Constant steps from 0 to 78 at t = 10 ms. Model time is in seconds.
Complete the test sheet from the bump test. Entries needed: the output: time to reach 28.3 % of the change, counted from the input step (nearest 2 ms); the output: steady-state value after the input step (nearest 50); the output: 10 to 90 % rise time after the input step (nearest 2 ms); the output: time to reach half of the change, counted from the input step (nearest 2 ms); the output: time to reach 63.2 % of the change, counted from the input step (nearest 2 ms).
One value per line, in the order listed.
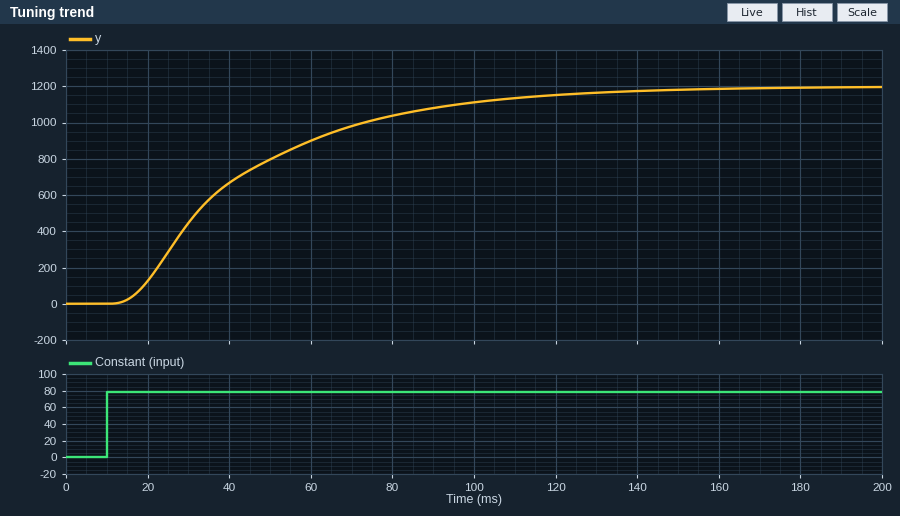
16 ms
1200
70 ms
26 ms
36 ms
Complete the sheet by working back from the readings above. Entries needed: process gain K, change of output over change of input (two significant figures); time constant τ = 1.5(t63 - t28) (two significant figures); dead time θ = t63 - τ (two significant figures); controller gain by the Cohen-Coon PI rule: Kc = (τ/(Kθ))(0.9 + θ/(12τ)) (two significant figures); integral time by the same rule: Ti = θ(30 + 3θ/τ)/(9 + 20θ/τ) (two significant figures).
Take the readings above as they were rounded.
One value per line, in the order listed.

15
30 ms
6.0 ms
0.31
14 ms
